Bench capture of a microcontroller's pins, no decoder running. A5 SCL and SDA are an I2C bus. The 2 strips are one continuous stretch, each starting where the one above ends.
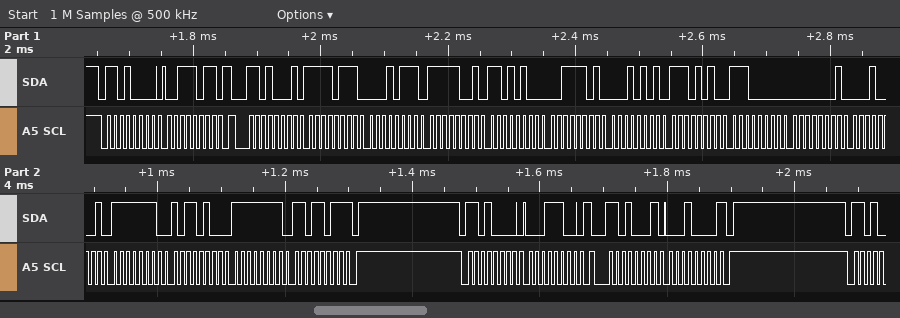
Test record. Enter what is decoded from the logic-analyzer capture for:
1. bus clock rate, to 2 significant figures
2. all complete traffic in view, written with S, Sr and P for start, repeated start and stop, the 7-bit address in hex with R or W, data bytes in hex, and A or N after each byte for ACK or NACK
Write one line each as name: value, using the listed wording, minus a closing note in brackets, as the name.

bus clock rate, to 2 significant figures: 100 kHz
all complete traffic in view, written with S, Sr and P for start, repeated start and stop, the 7-bit address in hex with R or W, data bytes in hex, and A or N after each byte for ACK or NACK: S 68W A 3B A Sr 68R A F7 A 17 A F9 A D4 A 3D A 15 A EA A E0 A 01 A 11 A FE A B4 A FF A DB N P S 68W A 1C A Sr 68R A 10 N P
